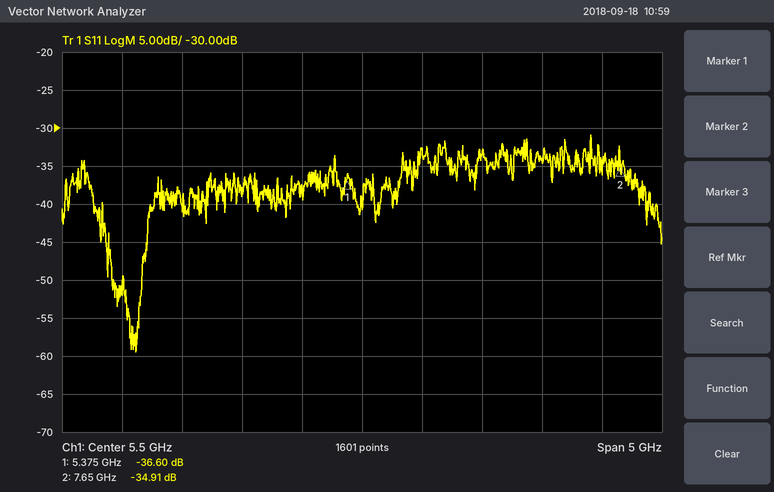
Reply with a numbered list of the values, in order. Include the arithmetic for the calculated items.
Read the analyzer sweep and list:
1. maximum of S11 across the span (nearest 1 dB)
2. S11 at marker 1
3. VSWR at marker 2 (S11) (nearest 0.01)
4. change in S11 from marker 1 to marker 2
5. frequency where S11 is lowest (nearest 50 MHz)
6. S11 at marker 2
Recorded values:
1. -31 dB
2. -36.60 dB
3. (1 + 0.0180)/(1 − 0.0180) ≈ 1.04
4. -34.91 − (-36.6) = 1.69 dB
5. 3.60 GHz
6. -34.91 dB
